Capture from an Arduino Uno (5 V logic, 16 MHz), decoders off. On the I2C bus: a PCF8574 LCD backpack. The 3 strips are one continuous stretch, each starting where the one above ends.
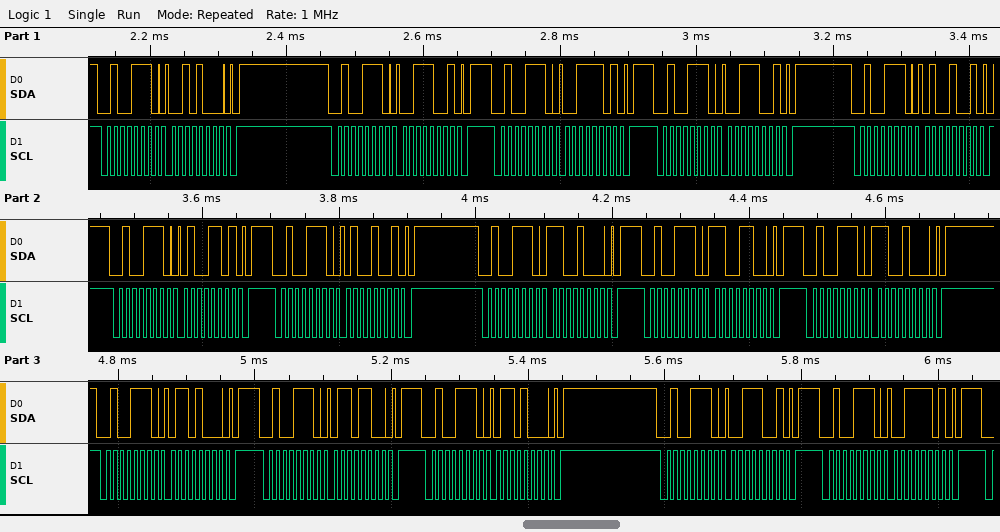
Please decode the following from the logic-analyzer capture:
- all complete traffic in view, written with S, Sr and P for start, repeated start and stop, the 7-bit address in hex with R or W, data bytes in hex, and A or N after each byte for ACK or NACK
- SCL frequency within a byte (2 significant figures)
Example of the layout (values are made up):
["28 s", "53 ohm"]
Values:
["S 27W A 28 A P S 27W A 39 A P S 27W A 3D A P S 27W A 39 A P S 27W A 49 A P S 27W A 4D A P S 27W A 49 A P S 27W A C8 A P S 27W A CC A P S 27W A C8 A P S 27W A 68 A P S 27W A 6C A P S 27W A 68 A P S 27W A 39 A P S 27W A 3D A P", "100 kHz"]
